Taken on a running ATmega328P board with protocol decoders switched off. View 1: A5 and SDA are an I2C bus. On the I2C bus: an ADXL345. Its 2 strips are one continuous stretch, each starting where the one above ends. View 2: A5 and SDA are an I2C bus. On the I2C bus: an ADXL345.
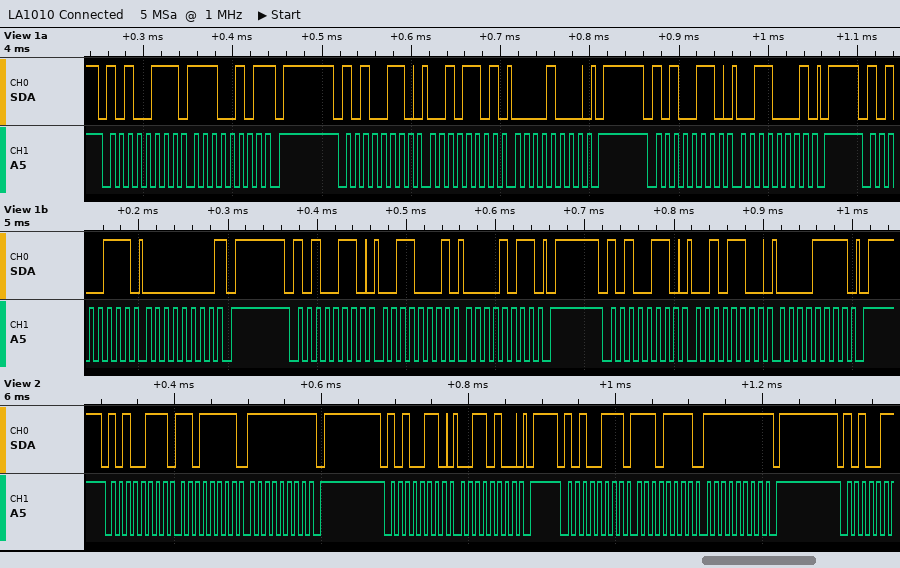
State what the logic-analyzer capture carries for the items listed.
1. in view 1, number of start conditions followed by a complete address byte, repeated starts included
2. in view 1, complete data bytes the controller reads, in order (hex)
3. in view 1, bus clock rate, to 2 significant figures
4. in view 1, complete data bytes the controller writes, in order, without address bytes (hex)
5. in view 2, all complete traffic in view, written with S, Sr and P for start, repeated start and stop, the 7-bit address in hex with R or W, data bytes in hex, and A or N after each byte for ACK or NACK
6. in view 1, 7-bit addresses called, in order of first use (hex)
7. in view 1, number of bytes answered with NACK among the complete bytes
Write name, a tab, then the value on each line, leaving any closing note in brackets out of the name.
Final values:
in view 1, number of start conditions followed by a complete address byte, repeated starts included	6
in view 1, complete data bytes the controller reads, in order	E5 00
in view 1, bus clock rate, to 2 significant figures	100 kHz
in view 1, complete data bytes the controller writes, in order, without address bytes	2D 08 31 31 0B 2C 0F
in view 2, all complete traffic in view, written with S, Sr and P for start, repeated start and stop, the 7-bit address in hex with R or W, data bytes in hex, and A or N after each byte for ACK or NACK	S 53R A DF A FF N P S 53W A 34 A P S 53R A EF A FF N P
in view 1, 7-bit addresses called, in order of first use	0x53
in view 1, number of bytes answered with NACK among the complete bytes	2
